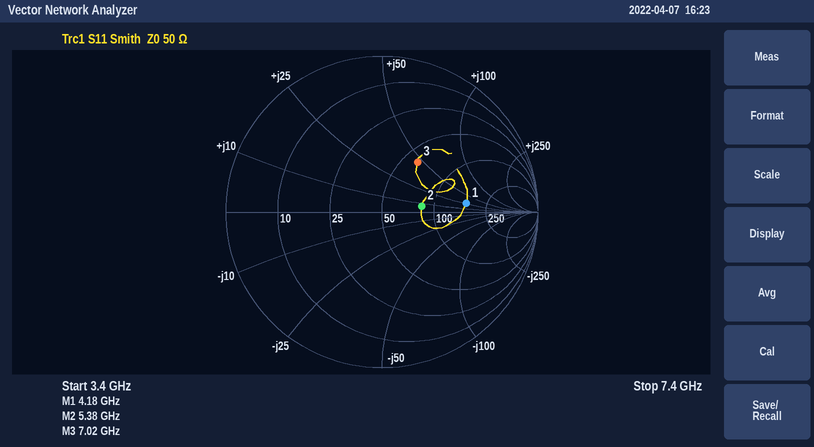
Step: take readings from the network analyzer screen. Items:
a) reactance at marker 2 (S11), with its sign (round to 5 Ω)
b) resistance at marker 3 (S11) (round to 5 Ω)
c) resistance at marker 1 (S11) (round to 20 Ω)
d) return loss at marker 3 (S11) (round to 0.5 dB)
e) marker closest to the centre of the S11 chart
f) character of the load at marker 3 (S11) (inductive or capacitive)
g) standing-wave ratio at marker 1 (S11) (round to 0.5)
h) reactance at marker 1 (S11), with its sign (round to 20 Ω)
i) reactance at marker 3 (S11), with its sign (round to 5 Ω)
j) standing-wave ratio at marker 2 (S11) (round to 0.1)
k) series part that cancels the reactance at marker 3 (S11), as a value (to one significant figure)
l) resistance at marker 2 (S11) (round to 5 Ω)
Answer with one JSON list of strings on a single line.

["+5 Ω", "60 Ω", "160 Ω", "8.0 dB", "marker 2", "inductive", "3.5", "+20 Ω", "+45 Ω", "1.7", "500 fF", "85 Ω"]
